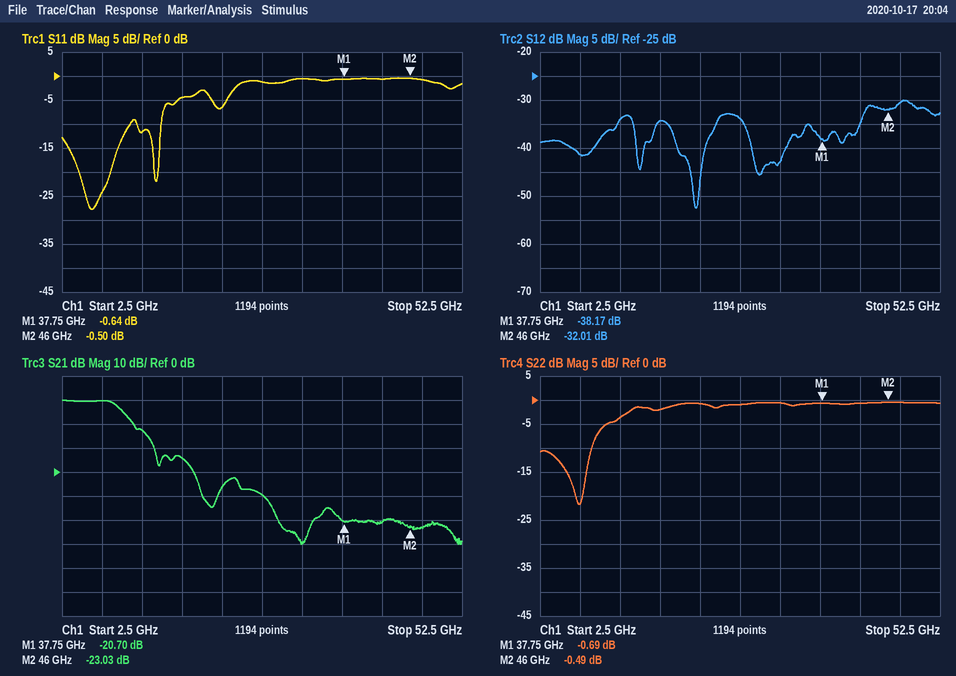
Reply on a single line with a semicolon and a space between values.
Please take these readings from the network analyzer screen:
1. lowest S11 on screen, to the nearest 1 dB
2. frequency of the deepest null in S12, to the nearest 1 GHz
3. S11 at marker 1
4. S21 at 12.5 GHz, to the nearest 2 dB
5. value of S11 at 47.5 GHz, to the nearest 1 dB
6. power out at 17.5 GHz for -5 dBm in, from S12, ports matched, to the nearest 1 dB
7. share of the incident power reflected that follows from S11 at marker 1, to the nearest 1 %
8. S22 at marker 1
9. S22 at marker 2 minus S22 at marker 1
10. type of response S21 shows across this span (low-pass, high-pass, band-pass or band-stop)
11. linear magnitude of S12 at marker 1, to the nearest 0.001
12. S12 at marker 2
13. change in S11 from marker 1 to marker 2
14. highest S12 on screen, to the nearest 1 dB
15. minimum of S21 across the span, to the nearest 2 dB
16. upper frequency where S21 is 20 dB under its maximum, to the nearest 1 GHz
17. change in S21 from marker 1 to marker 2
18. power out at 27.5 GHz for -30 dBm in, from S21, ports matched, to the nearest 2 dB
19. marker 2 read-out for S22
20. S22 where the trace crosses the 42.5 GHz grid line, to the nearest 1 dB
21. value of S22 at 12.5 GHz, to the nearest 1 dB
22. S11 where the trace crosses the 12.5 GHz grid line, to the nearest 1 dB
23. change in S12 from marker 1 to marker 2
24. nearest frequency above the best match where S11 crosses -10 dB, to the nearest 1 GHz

-28 dB; 22 GHz; -0.64 dB; 18 dB; -1 dB; -39 dBm; 86 %; -0.69 dB; 0.20 dB; low-pass; 0.012; -32.01 dB; 0.14 dB; -30 dB; -30 dB; 14 GHz; -2.33 dB; -40 dBm; -0.49 dB; -1 dB; -4 dB; -12 dB; 6.16 dB; 11 GHz
